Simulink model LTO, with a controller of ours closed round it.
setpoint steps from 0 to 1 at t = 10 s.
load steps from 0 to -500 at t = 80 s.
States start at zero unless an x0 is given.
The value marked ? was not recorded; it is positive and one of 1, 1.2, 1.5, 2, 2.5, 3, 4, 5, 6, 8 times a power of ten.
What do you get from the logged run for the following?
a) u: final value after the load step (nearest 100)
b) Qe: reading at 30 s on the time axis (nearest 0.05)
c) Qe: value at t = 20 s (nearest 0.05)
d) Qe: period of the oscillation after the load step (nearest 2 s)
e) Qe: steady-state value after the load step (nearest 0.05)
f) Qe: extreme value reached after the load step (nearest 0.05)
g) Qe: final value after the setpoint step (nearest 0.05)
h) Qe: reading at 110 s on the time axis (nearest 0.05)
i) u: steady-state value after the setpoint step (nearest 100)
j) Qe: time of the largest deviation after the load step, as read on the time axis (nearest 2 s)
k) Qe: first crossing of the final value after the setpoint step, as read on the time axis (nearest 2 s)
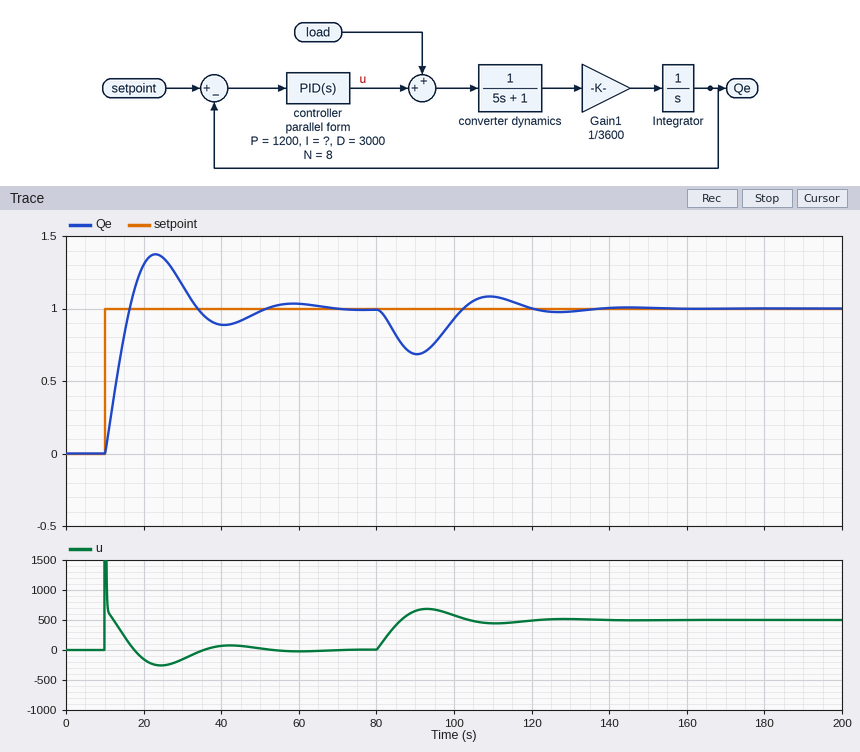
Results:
500
1.15
1.30
36 s
1.00
0.70
1.00
1.10
0
90 s
16 s
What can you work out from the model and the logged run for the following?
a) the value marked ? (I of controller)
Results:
150
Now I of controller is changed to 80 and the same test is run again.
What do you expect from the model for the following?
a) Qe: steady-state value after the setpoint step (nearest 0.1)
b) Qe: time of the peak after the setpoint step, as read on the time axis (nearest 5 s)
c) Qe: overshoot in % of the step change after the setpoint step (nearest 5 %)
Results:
1.0
25 s
25 %
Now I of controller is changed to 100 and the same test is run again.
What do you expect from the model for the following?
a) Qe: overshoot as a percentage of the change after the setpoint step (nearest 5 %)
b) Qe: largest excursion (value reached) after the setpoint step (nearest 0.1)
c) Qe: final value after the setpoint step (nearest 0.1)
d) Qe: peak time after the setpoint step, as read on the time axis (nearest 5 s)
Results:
30 %
1.3
1.0
25 s
